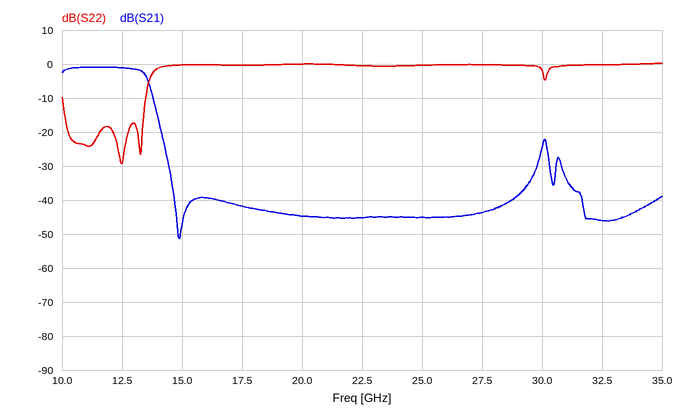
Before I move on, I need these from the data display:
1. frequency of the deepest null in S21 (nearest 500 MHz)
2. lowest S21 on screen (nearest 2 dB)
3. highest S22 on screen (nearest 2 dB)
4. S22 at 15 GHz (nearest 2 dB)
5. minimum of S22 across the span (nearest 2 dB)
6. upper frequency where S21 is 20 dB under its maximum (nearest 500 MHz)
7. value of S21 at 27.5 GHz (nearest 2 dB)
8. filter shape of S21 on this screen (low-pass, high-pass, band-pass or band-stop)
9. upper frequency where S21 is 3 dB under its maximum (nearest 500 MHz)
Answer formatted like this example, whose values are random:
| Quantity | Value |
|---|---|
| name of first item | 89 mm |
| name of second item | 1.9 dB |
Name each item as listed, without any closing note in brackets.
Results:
| Quantity | Value |
|---|---|
| frequency of the deepest null in S21 | 15.0 GHz |
| lowest S21 on screen | -52 dB |
| highest S22 on screen | 0 dB |
| S22 at 15 GHz | 0 dB |
| minimum of S22 across the span | -30 dB |
| upper frequency where S21 is 20 dB under its maximum | 14.0 GHz |
| value of S21 at 27.5 GHz | -44 dB |
| filter shape of S21 on this screen | low-pass |
| upper frequency where S21 is 3 dB under its maximum | 13.5 GHz |
